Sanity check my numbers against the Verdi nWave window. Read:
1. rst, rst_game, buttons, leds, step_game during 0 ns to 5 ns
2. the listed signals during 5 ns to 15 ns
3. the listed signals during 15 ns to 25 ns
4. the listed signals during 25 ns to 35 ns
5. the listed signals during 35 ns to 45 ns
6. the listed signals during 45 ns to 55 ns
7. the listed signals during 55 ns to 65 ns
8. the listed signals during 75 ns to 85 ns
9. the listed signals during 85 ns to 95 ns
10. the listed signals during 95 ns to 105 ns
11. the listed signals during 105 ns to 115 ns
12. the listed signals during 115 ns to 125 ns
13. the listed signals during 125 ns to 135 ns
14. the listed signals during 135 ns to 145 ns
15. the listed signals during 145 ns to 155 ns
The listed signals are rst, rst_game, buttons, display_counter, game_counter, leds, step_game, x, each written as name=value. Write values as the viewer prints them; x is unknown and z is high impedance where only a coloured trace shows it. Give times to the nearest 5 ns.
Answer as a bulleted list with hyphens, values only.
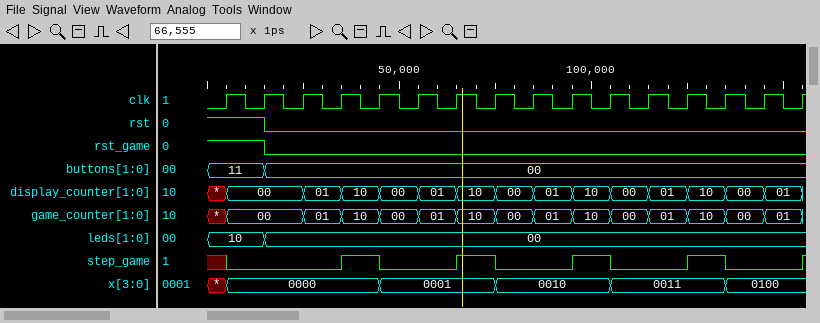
- rst=1, rst_game=1, buttons=11, leds=10, step_game=x
- rst=1, rst_game=1, buttons=11, display_counter=00, game_counter=00, leds=10, step_game=0, x=0000
- rst=0, rst_game=0, buttons=00, display_counter=00, game_counter=00, leds=00, step_game=0, x=0000
- rst=0, rst_game=0, buttons=00, display_counter=01, game_counter=01, leds=00, step_game=0, x=0000
- rst=0, rst_game=0, buttons=00, display_counter=10, game_counter=10, leds=00, step_game=1, x=0000
- rst=0, rst_game=0, buttons=00, display_counter=00, game_counter=00, leds=00, step_game=0, x=0001
- rst=0, rst_game=0, buttons=00, display_counter=01, game_counter=01, leds=00, step_game=0, x=0001
- rst=0, rst_game=0, buttons=00, display_counter=00, game_counter=00, leds=00, step_game=0, x=0010
- rst=0, rst_game=0, buttons=00, display_counter=01, game_counter=01, leds=00, step_game=0, x=0010
- rst=0, rst_game=0, buttons=00, display_counter=10, game_counter=10, leds=00, step_game=1, x=0010
- rst=0, rst_game=0, buttons=00, display_counter=00, game_counter=00, leds=00, step_game=0, x=0011
- rst=0, rst_game=0, buttons=00, display_counter=01, game_counter=01, leds=00, step_game=0, x=0011
- rst=0, rst_game=0, buttons=00, display_counter=10, game_counter=10, leds=00, step_game=1, x=0011
- rst=0, rst_game=0, buttons=00, display_counter=00, game_counter=00, leds=00, step_game=0, x=0100
- rst=0, rst_game=0, buttons=00, display_counter=01, game_counter=01, leds=00, step_game=0, x=0100
